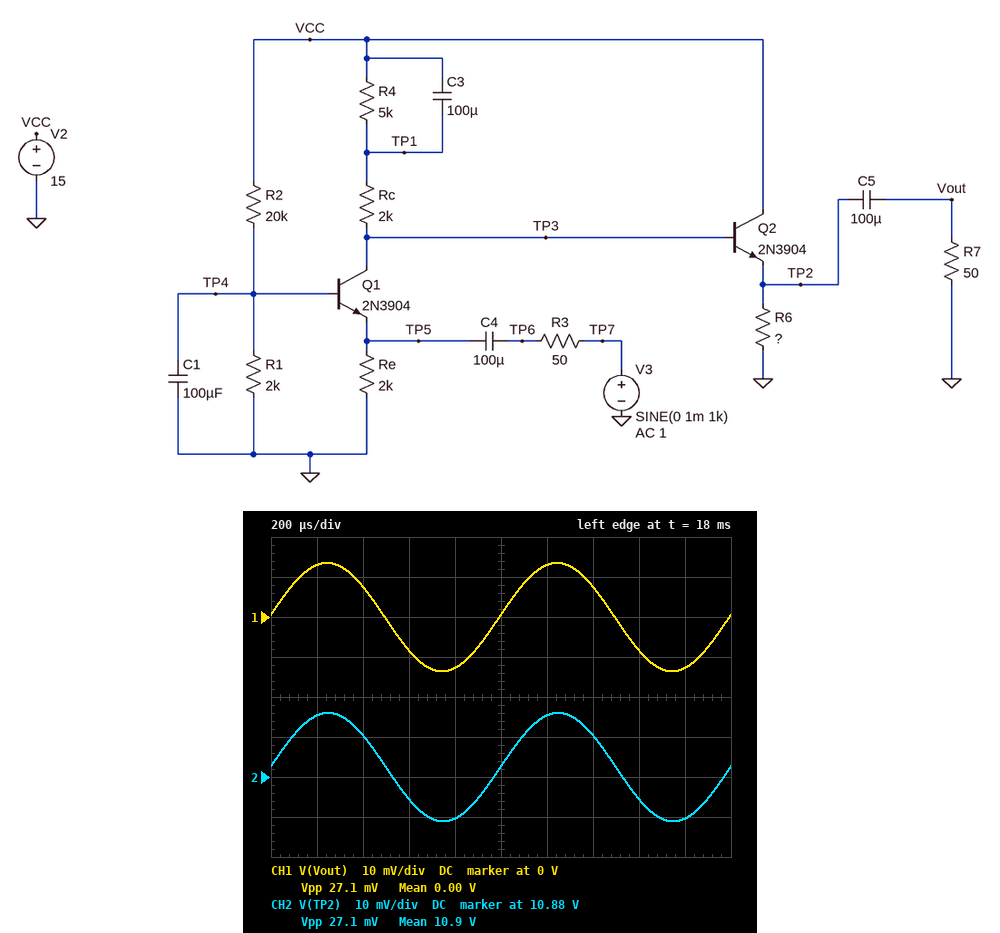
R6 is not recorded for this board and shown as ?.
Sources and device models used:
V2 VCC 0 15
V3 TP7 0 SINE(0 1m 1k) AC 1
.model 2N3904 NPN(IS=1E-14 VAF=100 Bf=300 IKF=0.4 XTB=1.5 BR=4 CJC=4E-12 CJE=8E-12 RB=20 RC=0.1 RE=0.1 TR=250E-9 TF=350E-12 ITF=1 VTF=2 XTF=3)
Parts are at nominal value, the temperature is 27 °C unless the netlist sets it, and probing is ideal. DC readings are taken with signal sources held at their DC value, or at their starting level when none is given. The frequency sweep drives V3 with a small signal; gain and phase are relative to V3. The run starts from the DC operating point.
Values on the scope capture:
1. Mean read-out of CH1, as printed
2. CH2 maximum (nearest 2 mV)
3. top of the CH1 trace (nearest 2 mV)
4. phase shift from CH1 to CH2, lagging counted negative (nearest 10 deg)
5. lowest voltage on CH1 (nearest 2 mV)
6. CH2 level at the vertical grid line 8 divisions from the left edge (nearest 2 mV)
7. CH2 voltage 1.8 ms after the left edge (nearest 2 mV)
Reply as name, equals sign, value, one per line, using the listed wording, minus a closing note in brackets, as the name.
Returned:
Mean read-out of CH1, as printed = 0.00 V
CH2 maximum = 10.896 V
top of the CH1 trace = 14 mV
phase shift from CH1 to CH2, lagging counted negative = 0 deg
lowest voltage on CH1 = -14 mV
CH2 level at the vertical grid line 8 divisions from the left edge = 10.874 V
CH2 voltage 1.8 ms after the left edge = 10.870 V
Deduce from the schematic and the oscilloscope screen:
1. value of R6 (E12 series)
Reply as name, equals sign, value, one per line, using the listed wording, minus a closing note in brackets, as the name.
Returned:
value of R6 = 330 Ω
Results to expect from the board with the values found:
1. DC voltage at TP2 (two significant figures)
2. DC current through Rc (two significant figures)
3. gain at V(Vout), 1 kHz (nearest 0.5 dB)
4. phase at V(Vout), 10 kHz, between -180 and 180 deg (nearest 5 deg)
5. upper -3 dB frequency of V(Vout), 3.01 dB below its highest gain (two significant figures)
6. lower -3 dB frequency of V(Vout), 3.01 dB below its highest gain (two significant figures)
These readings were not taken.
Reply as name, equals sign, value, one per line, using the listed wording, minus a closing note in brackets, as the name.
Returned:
DC voltage at TP2 = 11 V
DC current through Rc = 480 µA
gain at V(Vout), 1 kHz = 22.5 dB
phase at V(Vout), 10 kHz, between -180 and 180 deg = 0 deg
upper -3 dB frequency of V(Vout), 3.01 dB below its highest gain = 7.4 MHz
lower -3 dB frequency of V(Vout), 3.01 dB below its highest gain = 33 Hz
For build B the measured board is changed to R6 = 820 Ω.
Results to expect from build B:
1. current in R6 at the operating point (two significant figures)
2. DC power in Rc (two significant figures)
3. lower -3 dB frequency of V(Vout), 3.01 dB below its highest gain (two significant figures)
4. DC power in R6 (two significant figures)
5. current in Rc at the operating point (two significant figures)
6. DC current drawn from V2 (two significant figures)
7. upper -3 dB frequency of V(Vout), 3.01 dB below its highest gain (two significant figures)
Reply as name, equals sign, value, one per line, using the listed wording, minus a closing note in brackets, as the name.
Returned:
current in R6 at the operating point = 14 mA
DC power in Rc = 340 µW
lower -3 dB frequency of V(Vout), 3.01 dB below its highest gain = 32 Hz
DC power in R6 = 160 mW
current in Rc at the operating point = 410 µA
DC current drawn from V2 = 15 mA
upper -3 dB frequency of V(Vout), 3.01 dB below its highest gain = 7.5 MHz
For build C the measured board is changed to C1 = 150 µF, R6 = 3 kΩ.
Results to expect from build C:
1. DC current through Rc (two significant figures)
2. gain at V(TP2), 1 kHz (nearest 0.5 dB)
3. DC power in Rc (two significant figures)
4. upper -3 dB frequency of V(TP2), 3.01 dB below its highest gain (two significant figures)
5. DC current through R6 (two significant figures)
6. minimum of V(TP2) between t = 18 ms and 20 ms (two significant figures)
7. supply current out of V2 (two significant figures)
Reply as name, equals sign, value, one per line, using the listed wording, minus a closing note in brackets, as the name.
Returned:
DC current through Rc = 380 µA
gain at V(TP2), 1 kHz = 22.0 dB
DC power in Rc = 290 µW
upper -3 dB frequency of V(TP2), 3.01 dB below its highest gain = 6.9 MHz
DC current through R6 = 3.9 mA
minimum of V(TP2) between t = 18 ms and 20 ms = 12 V
supply current out of V2 = 4.9 mA
